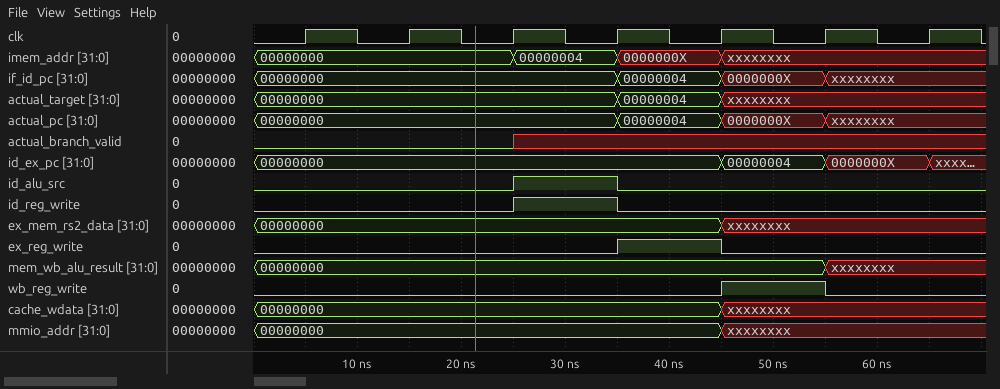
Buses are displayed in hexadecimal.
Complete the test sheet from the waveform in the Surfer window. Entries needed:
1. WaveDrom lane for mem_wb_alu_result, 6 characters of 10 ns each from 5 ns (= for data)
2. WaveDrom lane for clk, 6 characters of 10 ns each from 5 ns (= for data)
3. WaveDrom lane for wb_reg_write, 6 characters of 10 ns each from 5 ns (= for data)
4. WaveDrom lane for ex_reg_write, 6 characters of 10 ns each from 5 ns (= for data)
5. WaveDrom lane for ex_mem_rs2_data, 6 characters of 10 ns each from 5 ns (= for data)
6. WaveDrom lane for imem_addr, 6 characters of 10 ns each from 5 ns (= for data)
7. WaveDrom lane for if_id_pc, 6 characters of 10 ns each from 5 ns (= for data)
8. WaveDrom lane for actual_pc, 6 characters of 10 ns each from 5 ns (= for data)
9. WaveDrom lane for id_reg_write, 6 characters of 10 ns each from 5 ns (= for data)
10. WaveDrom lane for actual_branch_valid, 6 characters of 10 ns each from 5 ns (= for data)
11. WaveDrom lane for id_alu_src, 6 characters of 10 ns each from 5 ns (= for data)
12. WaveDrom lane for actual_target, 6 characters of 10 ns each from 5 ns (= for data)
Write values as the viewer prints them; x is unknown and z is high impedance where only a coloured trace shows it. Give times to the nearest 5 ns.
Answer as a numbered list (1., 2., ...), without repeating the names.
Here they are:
1. {name: 'mem_wb_alu_result', wave: '=....x', data: '00000000'}
2. {name: 'clk', wave: 'p.....'}
3. {name: 'wb_reg_write', wave: '0...10'}
4. {name: 'ex_reg_write', wave: '0..10.'}
5. {name: 'ex_mem_rs2_data', wave: '=...x.', data: '00000000'}
6. {name: 'imem_addr', wave: '=.==x.', data: '00000000 00000004 0000000X'}
7. {name: 'if_id_pc', wave: '=..==x', data: '00000000 00000004 0000000X'}
8. {name: 'actual_pc', wave: '=..==x', data: '00000000 00000004 0000000X'}
9. {name: 'id_reg_write', wave: '0.10..'}
10. {name: 'actual_branch_valid', wave: '0.x...'}
11. {name: 'id_alu_src', wave: '0.10..'}
12. {name: 'actual_target', wave: '=..=x.', data: '00000000 00000004'}
